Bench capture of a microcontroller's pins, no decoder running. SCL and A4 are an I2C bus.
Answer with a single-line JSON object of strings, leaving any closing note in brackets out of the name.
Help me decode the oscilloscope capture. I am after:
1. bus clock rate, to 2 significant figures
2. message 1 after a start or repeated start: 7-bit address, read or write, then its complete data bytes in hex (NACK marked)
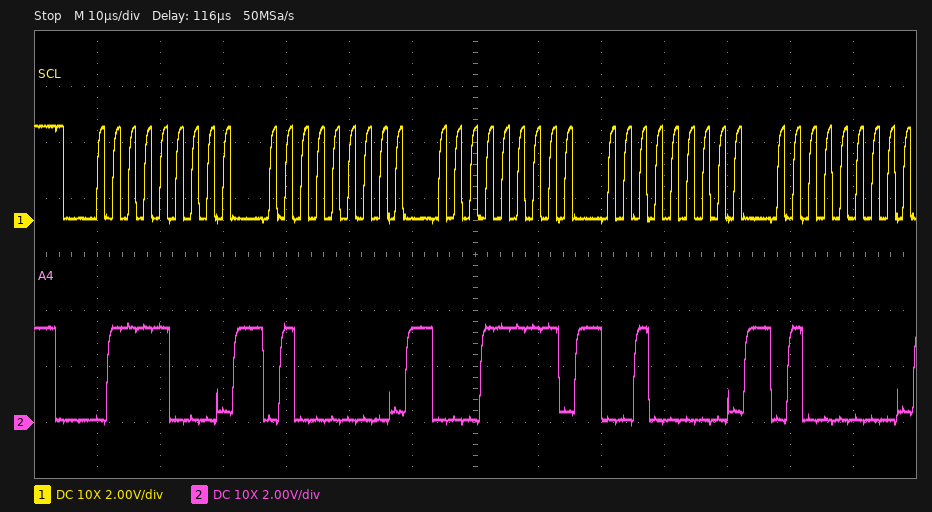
{"bus clock rate, to 2 significant figures": "400 kHz", "message 1 after a start or repeated start: 7-bit address, read or write, then its complete data bytes in hex": "0x3C write: 40 1F 20 40"}
